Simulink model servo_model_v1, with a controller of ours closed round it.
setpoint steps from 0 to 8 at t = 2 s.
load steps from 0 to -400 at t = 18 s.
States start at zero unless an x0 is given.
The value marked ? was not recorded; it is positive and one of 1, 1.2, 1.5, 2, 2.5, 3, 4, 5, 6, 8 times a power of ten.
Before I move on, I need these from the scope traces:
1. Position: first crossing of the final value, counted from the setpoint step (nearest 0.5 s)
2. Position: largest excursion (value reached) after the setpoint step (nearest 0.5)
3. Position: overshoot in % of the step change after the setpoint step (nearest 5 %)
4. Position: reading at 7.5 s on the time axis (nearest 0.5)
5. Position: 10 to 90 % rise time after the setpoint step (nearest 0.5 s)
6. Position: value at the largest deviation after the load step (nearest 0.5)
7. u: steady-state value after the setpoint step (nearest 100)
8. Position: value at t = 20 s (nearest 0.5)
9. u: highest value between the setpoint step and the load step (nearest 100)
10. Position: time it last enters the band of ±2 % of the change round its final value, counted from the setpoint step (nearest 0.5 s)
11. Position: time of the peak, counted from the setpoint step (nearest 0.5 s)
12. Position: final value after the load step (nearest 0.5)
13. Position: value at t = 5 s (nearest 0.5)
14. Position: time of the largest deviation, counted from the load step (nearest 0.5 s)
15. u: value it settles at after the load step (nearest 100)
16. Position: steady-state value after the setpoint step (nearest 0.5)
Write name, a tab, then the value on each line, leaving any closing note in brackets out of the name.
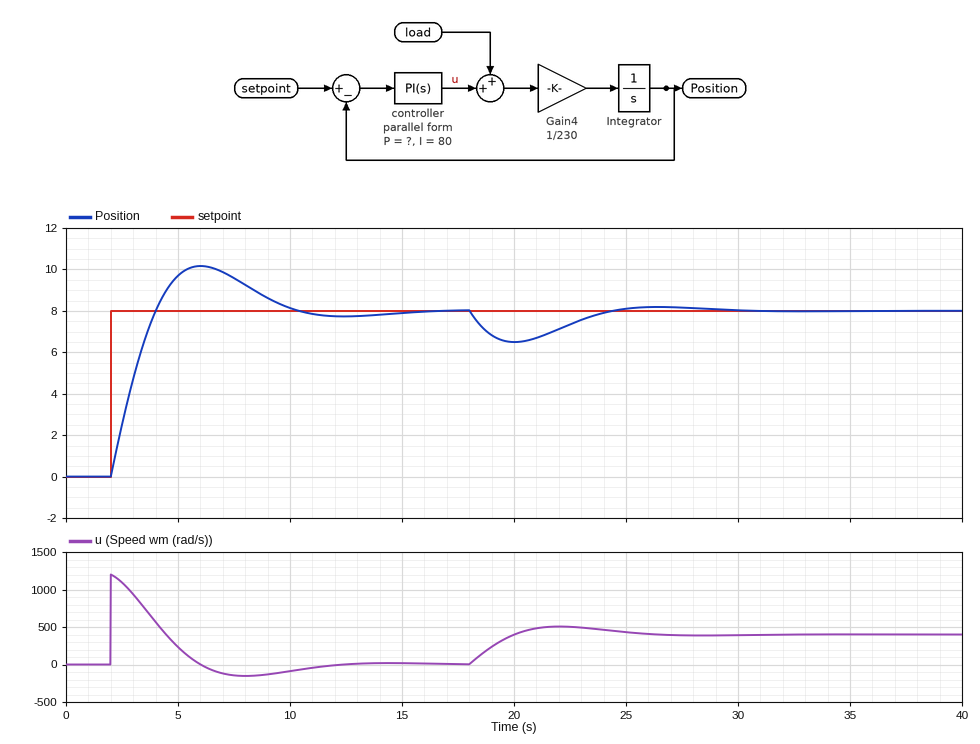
Position: first crossing of the final value, counted from the setpoint step	2.0 s
Position: largest excursion (value reached) after the setpoint step	10.0
Position: overshoot in % of the step change after the setpoint step	25 %
Position: reading at 7.5 s on the time axis	9.5
Position: 10 to 90 % rise time after the setpoint step	1.5 s
Position: value at the largest deviation after the load step	6.5
u: steady-state value after the setpoint step	0
Position: value at t = 20 s	6.5
u: highest value between the setpoint step and the load step	1200
Position: time it last enters the band of ±2 % of the change round its final value, counted from the setpoint step	12.5 s
Position: time of the peak, counted from the setpoint step	4.0 s
Position: final value after the load step	8.0
Position: value at t = 5 s	9.5
Position: time of the largest deviation, counted from the load step	2.0 s
u: value it settles at after the load step	400
Position: steady-state value after the setpoint step	8.0
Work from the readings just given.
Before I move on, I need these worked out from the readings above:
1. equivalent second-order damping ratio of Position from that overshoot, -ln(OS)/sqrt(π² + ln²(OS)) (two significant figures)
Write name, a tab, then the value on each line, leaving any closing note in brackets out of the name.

equivalent second-order damping ratio of Position from that overshoot, -ln(OS)/sqrt(π² + ln²(OS))	0.40
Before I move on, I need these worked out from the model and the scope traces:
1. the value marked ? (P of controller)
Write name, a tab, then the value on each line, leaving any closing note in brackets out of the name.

the value marked ?	150
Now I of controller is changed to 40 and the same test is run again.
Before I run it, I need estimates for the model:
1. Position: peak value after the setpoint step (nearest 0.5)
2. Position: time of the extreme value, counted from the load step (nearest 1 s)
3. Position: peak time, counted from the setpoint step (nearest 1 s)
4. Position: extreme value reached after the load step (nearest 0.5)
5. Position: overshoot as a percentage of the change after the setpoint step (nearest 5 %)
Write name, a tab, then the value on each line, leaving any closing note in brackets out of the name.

Position: peak value after the setpoint step	9.5
Position: time of the extreme value, counted from the load step	3 s
Position: peak time, counted from the setpoint step	5 s
Position: extreme value reached after the load step	6.0
Position: overshoot as a percentage of the change after the setpoint step	20 %
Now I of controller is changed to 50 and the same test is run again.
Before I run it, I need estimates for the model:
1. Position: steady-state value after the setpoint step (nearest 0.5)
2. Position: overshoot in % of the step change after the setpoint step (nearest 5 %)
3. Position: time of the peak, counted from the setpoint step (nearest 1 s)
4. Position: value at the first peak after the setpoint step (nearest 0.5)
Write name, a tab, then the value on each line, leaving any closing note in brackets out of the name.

Position: steady-state value after the setpoint step	8.0
Position: overshoot in % of the step change after the setpoint step	20 %
Position: time of the peak, counted from the setpoint step	5 s
Position: value at the first peak after the setpoint step	9.5
